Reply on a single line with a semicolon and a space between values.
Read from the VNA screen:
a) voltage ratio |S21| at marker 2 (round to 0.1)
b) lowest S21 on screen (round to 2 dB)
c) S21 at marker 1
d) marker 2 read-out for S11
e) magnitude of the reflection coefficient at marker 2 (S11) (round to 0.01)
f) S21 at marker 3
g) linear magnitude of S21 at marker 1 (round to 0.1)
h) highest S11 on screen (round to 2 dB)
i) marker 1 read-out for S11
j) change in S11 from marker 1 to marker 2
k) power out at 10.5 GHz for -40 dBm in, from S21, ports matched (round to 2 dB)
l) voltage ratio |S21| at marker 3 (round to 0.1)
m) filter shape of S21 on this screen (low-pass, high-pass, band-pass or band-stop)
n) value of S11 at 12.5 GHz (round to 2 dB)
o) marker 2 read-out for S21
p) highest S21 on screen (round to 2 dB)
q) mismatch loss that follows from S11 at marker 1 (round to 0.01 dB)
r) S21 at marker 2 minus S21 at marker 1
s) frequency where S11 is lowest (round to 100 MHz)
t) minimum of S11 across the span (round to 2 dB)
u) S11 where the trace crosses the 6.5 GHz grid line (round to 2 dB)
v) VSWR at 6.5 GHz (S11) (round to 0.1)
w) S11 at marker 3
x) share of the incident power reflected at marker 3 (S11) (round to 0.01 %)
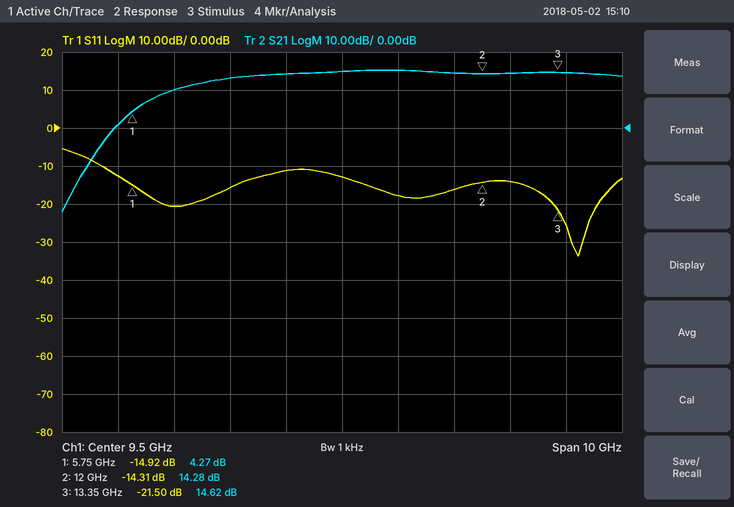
5.2; -22 dB; 4.27 dB; -14.31 dB; 0.19; 14.62 dB; 1.6; -6 dB; -14.92 dB; 0.61 dB; -24 dBm; 5.4; high-pass; -14 dB; 14.28 dB; 16 dB; 0.14 dB; 10.01 dB; 13.7 GHz; -34 dB; -20 dB; 1.2; -21.50 dB; 0.71 %
